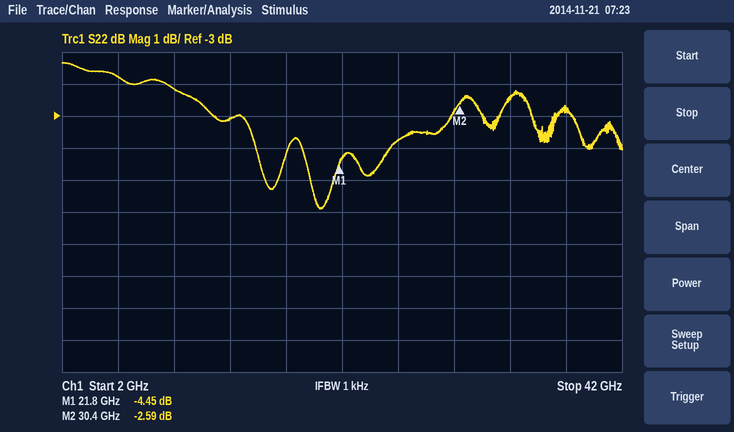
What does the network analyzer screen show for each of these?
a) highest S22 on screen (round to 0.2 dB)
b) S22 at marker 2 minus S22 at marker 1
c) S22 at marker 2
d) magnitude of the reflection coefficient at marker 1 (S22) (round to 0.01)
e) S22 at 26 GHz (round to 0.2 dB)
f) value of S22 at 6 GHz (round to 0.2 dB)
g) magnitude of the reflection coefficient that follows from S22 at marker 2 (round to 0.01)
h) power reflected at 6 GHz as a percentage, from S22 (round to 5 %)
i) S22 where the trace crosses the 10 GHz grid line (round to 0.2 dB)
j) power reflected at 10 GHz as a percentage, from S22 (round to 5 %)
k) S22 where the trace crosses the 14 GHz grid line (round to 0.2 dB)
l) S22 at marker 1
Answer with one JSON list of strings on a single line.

["-1.4 dB", "1.86 dB", "-2.59 dB", "0.60", "-3.8 dB", "-1.8 dB", "0.74", "65 %", "-2.2 dB", "60 %", "-3.0 dB", "-4.45 dB"]
